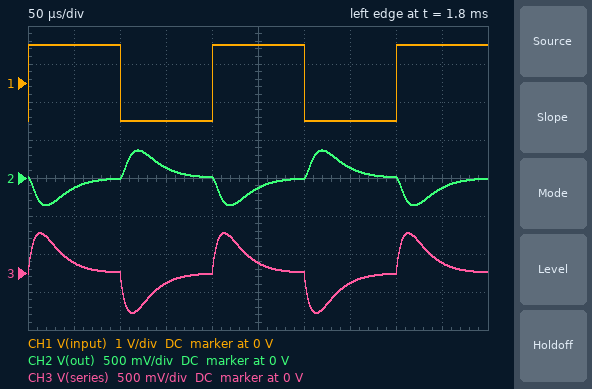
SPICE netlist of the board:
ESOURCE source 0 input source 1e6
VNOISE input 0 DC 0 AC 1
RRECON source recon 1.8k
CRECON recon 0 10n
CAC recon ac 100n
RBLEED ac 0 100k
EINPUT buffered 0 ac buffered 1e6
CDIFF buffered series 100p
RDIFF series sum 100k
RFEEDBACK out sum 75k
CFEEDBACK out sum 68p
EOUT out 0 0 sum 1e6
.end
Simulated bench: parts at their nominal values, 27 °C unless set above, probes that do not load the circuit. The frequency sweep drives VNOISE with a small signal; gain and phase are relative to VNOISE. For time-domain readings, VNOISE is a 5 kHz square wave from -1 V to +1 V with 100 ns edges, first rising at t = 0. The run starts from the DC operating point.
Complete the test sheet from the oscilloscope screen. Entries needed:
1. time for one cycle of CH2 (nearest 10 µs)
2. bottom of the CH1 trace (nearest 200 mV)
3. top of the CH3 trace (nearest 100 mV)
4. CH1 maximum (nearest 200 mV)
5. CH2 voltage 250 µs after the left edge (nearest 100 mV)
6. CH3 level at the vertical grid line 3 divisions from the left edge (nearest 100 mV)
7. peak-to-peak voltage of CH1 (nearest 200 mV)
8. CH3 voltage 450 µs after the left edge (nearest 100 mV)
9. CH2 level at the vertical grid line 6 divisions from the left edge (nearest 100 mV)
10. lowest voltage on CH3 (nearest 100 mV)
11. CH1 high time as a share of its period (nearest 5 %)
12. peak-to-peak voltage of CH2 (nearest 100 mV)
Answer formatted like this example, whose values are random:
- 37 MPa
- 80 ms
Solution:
- 200 µs
- -1.0 V
- 500 mV
- 1.0 V
- -100 mV
- -100 mV
- 2.0 V
- 100 mV
- 0 V
- -500 mV
- 50 %
- 700 mV
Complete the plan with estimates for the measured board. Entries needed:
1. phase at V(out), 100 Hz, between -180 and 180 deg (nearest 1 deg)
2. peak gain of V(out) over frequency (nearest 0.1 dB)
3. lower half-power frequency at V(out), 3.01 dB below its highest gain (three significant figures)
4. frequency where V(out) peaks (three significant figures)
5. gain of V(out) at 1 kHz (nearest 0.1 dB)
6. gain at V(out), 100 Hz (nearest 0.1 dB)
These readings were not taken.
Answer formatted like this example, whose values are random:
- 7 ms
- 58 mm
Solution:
- -82 deg
- -12.0 dB
- 4.48 kHz
- 10.7 kHz
- -26.8 dB
- -46.8 dB
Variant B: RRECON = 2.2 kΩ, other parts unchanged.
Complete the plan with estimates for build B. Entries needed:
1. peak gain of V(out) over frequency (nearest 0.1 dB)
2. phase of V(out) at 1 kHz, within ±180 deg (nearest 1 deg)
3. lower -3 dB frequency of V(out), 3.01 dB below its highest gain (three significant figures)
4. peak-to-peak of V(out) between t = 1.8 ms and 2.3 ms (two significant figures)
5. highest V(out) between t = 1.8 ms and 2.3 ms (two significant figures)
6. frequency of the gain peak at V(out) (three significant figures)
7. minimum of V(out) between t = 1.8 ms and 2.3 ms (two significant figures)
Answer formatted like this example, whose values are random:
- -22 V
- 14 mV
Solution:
- -13.1 dB
- -102 deg
- 4.01 kHz
- 640 mV
- 320 mV
- 9.78 kHz
- -320 mV
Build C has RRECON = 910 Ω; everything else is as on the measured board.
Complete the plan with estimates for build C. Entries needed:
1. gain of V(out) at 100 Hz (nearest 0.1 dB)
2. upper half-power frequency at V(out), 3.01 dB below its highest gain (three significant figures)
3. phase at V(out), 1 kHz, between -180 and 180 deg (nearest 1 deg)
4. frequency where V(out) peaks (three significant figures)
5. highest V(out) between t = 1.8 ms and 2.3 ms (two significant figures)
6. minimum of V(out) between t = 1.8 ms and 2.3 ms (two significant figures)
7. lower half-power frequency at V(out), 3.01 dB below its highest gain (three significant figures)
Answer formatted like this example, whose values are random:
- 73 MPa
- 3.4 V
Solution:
- -46.7 dB
- 29.0 kHz
- -98 deg
- 14.1 kHz
- 500 mV
- -500 mV
- 6.15 kHz
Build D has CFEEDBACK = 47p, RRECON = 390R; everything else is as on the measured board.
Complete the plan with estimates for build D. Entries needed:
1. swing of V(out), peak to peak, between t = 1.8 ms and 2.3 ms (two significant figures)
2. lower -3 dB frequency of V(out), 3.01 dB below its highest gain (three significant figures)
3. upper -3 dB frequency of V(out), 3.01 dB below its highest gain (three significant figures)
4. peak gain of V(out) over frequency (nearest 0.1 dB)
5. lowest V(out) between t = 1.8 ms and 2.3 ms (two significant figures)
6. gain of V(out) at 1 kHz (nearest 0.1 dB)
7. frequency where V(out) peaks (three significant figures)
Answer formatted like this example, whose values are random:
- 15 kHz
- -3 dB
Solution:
- 1.4 V
- 8.54 kHz
- 44.4 kHz
- -6.4 dB
- -700 mV
- -26.6 dB
- 20.6 kHz
